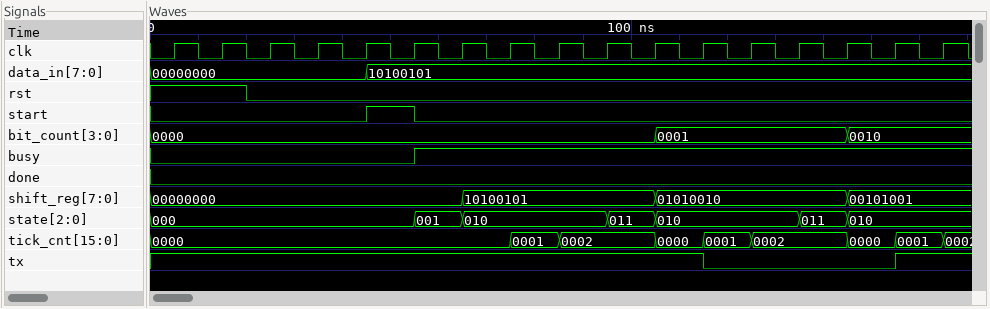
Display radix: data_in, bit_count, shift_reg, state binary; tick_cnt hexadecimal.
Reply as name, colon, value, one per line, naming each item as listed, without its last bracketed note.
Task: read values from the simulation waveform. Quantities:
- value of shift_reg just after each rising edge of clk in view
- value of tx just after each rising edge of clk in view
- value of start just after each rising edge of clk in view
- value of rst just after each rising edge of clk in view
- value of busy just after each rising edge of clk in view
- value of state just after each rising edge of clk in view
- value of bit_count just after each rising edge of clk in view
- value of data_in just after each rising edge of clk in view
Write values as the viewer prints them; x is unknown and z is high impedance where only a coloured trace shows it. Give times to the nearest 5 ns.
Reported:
value of shift_reg just after each rising edge of clk in view: 00000000, 00000000, 00000000, 00000000, 00000000, 00000000, 10100101, 10100101, 10100101, 10100101, 01010010, 01010010, 01010010, 01010010, 00101001, 00101001, 00101001
value of tx just after each rising edge of clk in view: 1 1 1 1 1 1 1 1 1 1 1 0 0 0 0 1 1
value of start just after each rising edge of clk in view: 0 0 0 0 1 0 0 0 0 0 0 0 0 0 0 0 0
value of rst just after each rising edge of clk in view: 1 1 0 0 0 0 0 0 0 0 0 0 0 0 0 0 0
value of busy just after each rising edge of clk in view: 0 0 0 0 0 1 1 1 1 1 1 1 1 1 1 1 1
value of state just after each rising edge of clk in view: 000, 000, 000, 000, 000, 001, 010, 010, 010, 011, 010, 010, 010, 011, 010, 010, 010
value of bit_count just after each rising edge of clk in view: 0000, 0000, 0000, 0000, 0000, 0000, 0000, 0000, 0000, 0000, 0001, 0001, 0001, 0001, 0010, 0010, 0010
value of data_in just after each rising edge of clk in view: 00000000, 00000000, 00000000, 00000000, 10100101, 10100101, 10100101, 10100101, 10100101, 10100101, 10100101, 10100101, 10100101, 10100101, 10100101, 10100101, 10100101
